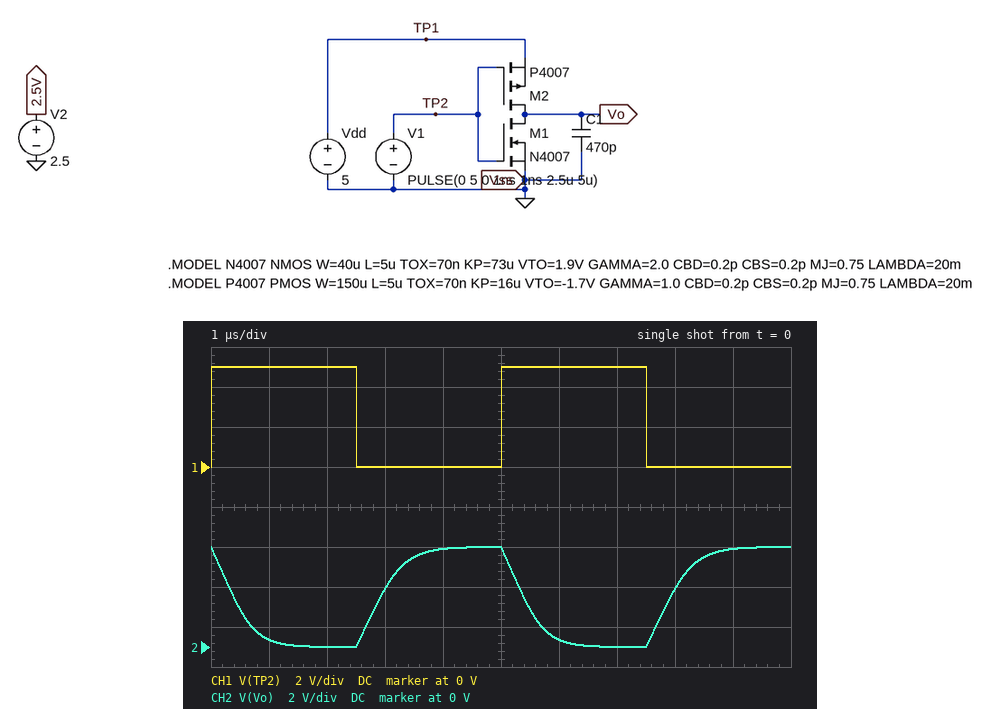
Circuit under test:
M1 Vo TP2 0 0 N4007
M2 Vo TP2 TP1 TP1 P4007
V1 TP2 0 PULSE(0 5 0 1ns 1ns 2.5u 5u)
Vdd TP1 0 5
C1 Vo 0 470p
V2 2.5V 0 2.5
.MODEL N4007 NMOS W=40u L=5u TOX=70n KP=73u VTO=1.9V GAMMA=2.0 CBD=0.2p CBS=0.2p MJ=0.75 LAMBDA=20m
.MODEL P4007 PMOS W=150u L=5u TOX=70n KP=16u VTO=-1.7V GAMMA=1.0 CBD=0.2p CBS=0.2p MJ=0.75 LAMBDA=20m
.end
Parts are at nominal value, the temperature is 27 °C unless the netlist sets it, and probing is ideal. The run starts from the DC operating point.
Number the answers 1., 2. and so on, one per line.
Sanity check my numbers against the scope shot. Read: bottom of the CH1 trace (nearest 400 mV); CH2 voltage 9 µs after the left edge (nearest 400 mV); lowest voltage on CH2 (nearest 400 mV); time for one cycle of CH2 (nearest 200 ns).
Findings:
1. 0 V
2. 4.8 V
3. 0 V
4. 5.0 µs
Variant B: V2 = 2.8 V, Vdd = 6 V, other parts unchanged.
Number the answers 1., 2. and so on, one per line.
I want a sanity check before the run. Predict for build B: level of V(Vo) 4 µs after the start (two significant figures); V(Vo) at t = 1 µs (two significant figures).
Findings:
1. 6.0 V
2. 620 mV
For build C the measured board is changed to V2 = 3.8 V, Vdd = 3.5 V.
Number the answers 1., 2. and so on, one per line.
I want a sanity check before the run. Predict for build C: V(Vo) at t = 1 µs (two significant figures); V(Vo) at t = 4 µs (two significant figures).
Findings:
1. 150 mV
2. 2.5 V
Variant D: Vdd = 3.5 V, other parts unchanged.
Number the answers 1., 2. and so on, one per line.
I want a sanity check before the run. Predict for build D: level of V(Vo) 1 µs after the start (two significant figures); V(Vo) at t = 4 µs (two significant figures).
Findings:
1. 150 mV
2. 2.5 V
